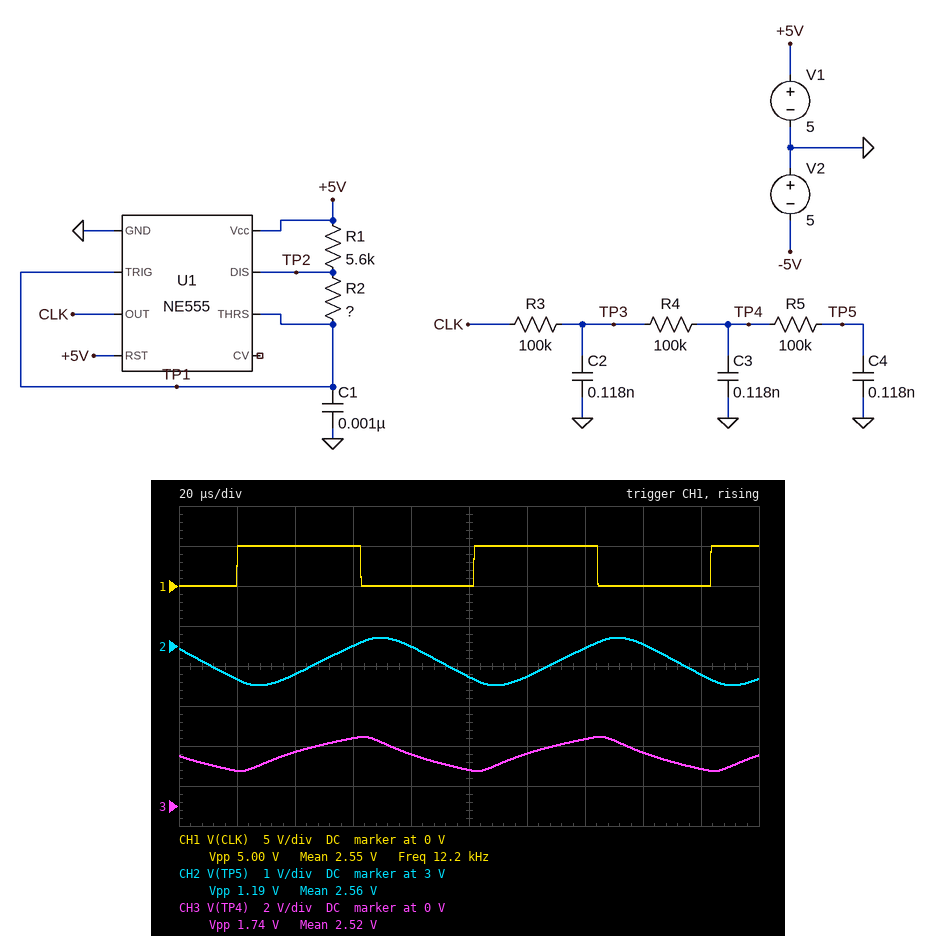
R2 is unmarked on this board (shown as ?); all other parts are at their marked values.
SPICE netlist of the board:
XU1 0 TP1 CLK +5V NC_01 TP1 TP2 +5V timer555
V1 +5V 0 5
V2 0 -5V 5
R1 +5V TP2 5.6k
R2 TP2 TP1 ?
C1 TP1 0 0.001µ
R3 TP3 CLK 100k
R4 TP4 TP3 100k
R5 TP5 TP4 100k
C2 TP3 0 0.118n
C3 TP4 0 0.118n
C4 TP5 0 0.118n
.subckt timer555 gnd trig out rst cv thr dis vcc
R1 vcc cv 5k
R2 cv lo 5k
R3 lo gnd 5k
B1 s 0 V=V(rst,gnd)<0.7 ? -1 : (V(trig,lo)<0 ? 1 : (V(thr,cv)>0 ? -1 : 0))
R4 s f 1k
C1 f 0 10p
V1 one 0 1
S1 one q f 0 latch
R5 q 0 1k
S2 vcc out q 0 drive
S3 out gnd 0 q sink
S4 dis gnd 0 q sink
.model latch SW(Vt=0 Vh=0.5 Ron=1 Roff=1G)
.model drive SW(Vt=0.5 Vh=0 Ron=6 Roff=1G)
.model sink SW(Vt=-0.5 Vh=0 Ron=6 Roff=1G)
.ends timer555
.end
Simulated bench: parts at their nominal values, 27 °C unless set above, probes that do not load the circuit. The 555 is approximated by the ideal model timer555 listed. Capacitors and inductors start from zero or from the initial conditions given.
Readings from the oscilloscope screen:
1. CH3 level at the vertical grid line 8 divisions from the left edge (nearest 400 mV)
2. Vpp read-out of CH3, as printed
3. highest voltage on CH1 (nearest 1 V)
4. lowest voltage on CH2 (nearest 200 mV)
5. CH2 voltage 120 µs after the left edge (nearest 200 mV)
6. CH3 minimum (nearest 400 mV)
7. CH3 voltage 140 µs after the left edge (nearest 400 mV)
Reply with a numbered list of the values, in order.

1. 2.8 V
2. 1.74 V
3. 5 V
4. 2.0 V
5. 2.2 V
6. 1.6 V
7. 3.2 V
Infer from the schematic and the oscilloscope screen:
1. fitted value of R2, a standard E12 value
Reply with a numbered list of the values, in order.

1. 56 kΩ
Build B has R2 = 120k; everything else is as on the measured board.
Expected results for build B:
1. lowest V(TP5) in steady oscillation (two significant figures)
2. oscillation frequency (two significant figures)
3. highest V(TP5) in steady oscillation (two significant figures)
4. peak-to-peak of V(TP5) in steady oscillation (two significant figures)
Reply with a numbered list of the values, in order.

1. 1.2 V
2. 5.9 kHz
3. 3.9 V
4. 2.8 V
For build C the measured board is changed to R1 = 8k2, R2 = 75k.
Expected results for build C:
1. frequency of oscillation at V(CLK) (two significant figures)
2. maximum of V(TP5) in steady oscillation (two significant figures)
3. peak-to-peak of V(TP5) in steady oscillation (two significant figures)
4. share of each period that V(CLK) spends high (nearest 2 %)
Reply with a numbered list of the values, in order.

1. 9.1 kHz
2. 3.5 V
3. 1.7 V
4. 52 %
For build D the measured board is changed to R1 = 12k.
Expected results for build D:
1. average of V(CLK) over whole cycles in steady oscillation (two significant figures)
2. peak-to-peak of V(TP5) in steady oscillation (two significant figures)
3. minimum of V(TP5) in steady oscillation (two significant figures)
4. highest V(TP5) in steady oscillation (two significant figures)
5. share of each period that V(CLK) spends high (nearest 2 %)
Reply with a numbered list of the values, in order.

1. 2.7 V
2. 1.3 V
3. 2.1 V
4. 3.4 V
5. 54 %
